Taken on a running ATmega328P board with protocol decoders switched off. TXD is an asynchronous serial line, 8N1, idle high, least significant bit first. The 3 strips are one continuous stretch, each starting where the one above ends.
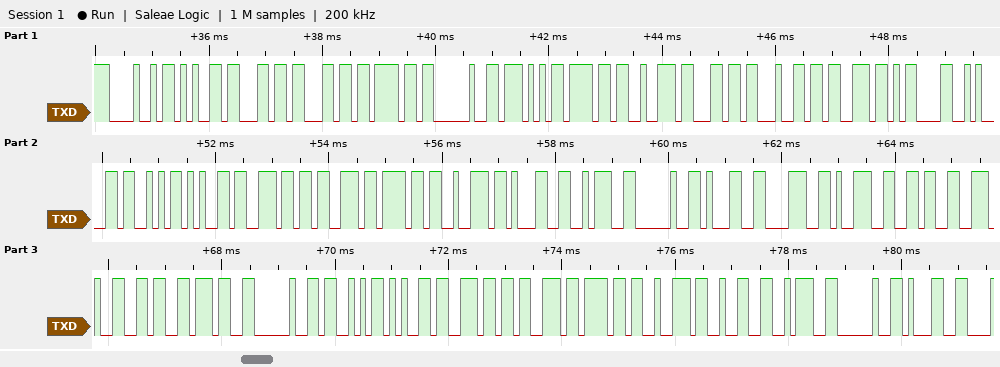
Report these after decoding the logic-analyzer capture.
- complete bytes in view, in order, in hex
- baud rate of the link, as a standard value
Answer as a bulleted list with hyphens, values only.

- 0x48 0x65 0x6C 0x6C 0x6F 0x20 0x57 0x6F 0x72 0x6C 0x64 0x73 0x0D 0x0A 0x53 0x65 0x6E 0x73 0x6F 0x72 0x31 0x3A 0x20 0x31 0x38 0x39 0x36 0x2E 0x36 0x37 0x20 0x53 0x65 0x6E 0x73 0x6F 0x72 0x32 0x3A 0x20 0x31
- 9600 baud
